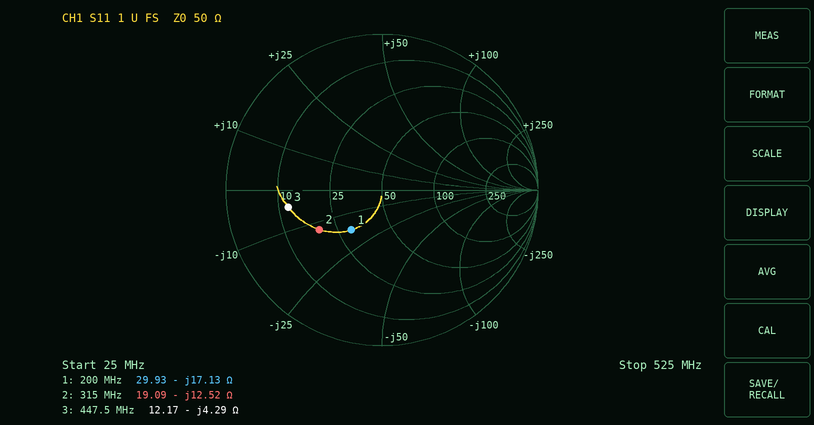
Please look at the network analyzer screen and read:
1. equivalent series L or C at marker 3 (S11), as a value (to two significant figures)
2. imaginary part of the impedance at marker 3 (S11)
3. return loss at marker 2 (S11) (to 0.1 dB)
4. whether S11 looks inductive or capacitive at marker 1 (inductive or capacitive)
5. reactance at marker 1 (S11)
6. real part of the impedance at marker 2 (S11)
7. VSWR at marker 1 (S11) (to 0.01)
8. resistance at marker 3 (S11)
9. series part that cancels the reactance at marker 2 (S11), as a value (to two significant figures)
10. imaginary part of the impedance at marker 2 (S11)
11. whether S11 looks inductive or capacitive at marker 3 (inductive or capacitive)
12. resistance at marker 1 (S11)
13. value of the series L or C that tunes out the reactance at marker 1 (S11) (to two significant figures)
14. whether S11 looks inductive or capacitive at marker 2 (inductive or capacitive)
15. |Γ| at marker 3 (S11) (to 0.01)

83 pF
-4.29 Ω
6.5 dB
capacitive
-17.13 Ω
19.09 Ω
1.95
12.17 Ω
6.3 nH
-12.52 Ω
capacitive
29.93 Ω
14 nH
capacitive
0.61
